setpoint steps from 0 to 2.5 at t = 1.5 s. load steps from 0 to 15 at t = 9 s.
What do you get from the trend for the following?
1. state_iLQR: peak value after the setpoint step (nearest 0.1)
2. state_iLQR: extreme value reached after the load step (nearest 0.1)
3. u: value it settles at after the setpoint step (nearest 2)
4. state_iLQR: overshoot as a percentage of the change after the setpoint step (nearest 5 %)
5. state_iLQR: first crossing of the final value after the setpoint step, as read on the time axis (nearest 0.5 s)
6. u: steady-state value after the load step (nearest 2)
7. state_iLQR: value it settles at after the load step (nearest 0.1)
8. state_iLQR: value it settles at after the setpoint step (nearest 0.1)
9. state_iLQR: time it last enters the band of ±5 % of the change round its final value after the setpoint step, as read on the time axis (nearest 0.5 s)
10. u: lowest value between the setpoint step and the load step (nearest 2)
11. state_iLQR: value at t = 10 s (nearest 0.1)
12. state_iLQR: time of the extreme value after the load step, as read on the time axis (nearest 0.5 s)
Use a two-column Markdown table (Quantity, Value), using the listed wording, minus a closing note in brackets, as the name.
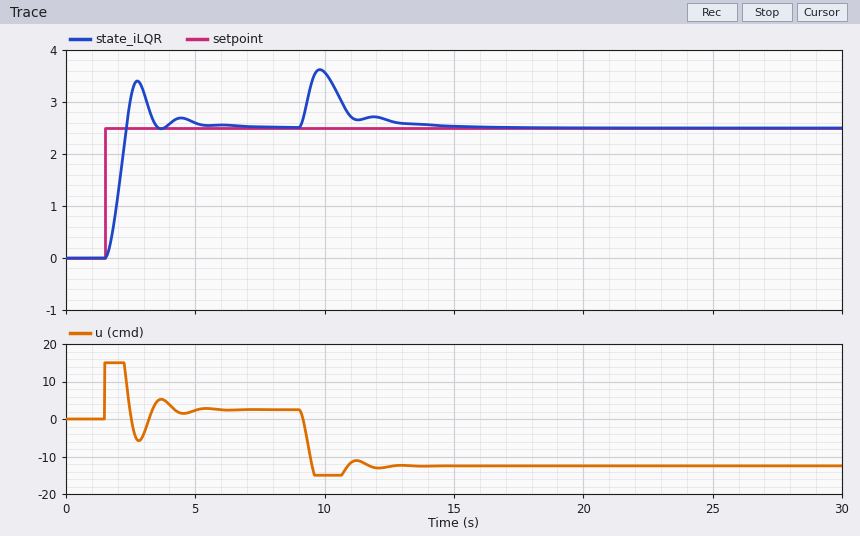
| Quantity | Value |
|---|---|
| state_iLQR: peak value after the setpoint step | 3.4 |
| state_iLQR: extreme value reached after the load step | 3.6 |
| u: value it settles at after the setpoint step | 2 |
| state_iLQR: overshoot as a percentage of the change after the setpoint step | 35 % |
| state_iLQR: first crossing of the final value after the setpoint step, as read on the time axis | 2.5 s |
| u: steady-state value after the load step | -12 |
| state_iLQR: value it settles at after the load step | 2.5 |
| state_iLQR: value it settles at after the setpoint step | 2.5 |
| state_iLQR: time it last enters the band of ±5 % of the change round its final value after the setpoint step, as read on the time axis | 5.0 s |
| u: lowest value between the setpoint step and the load step | -6 |
| state_iLQR: value at t = 10 s | 3.6 |
| state_iLQR: time of the extreme value after the load step, as read on the time axis | 10.0 s |
